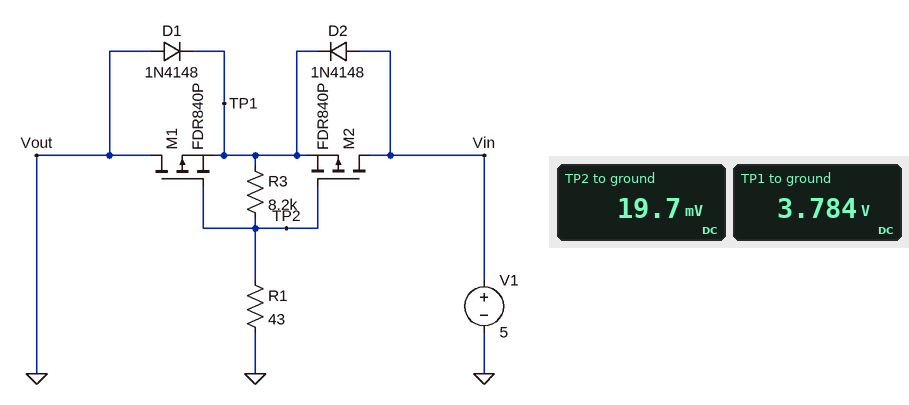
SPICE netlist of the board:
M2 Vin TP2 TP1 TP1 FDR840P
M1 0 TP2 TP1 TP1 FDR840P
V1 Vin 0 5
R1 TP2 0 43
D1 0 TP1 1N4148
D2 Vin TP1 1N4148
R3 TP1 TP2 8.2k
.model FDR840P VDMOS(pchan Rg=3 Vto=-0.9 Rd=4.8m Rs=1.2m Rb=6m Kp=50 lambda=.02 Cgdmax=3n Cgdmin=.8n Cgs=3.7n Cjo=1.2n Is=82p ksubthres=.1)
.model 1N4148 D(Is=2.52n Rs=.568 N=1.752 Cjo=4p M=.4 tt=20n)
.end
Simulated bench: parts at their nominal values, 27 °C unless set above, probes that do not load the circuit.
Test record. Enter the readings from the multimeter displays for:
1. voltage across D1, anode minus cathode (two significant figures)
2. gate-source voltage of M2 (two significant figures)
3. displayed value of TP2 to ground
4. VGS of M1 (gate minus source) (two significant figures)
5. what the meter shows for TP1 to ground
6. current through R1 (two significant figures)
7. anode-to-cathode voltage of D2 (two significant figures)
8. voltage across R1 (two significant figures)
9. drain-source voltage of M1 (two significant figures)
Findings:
-3.8 V
-3.8 V
19.7 mV
-3.8 V
3.784 V
460 µA
1.2 V
20 mV
-3.8 V
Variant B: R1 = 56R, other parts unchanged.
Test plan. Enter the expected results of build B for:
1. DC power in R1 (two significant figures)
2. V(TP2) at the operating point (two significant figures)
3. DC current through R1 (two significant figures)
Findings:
12 µW
26 mV
460 µA
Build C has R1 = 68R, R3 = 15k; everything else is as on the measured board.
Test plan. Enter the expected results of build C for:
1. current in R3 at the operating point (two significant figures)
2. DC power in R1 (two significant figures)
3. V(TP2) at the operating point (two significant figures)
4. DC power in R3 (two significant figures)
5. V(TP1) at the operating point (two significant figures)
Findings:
250 µA
4.3 µW
17 mV
950 µW
3.8 V
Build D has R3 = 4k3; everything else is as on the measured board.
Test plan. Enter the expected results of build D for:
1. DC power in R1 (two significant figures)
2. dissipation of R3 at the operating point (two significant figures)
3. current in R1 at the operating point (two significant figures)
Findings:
33 µW
3.3 mW
870 µA
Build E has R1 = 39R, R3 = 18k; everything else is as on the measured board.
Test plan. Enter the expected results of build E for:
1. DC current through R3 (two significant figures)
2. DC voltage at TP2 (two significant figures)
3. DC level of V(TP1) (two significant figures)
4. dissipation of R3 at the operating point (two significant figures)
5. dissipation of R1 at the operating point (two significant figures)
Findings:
210 µA
8.2 mV
3.8 V
790 µW
1.7 µW
